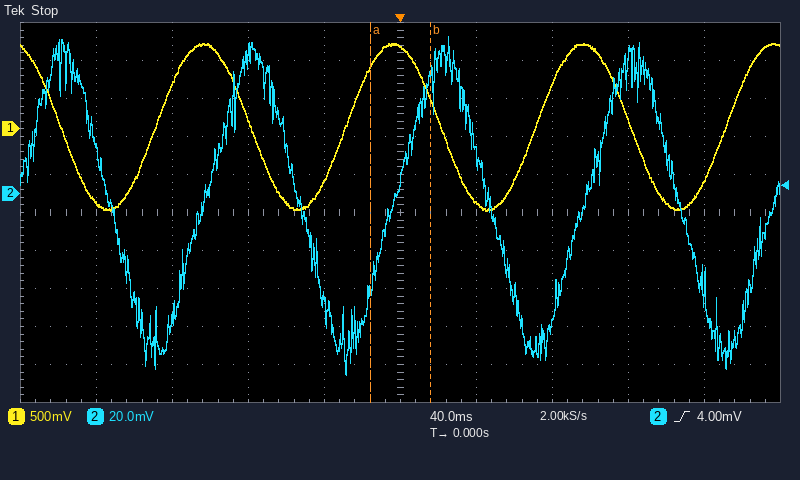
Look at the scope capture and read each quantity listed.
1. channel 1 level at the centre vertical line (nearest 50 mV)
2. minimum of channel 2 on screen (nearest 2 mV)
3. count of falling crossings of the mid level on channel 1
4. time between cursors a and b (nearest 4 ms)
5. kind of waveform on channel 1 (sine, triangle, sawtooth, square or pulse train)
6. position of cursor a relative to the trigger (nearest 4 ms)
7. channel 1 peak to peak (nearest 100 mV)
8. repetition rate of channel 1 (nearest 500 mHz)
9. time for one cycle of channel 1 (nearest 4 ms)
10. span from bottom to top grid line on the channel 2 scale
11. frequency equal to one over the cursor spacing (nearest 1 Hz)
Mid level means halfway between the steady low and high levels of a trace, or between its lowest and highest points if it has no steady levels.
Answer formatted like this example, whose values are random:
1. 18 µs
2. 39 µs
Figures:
1. 1.10 V
2. -96 mV
3. 4
4. 32 ms
5. sine
6. -16 ms
7. 2.20 V
8. 10.0 Hz
9. 100 ms
10. 200 mV
11. 31 Hz
